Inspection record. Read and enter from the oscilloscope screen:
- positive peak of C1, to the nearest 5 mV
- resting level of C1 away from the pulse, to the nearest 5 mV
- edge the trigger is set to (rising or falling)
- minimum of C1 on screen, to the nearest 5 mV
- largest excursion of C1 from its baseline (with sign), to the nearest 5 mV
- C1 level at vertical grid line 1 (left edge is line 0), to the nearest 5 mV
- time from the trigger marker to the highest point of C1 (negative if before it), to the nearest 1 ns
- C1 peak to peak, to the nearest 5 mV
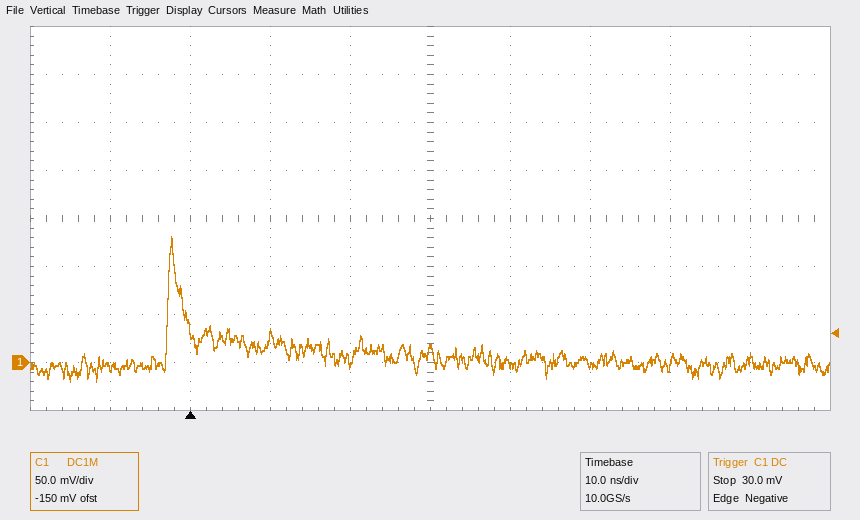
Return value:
130 mV
0 mV
falling
-20 mV
+130 mV
-5 mV
-2 ns
150 mV
